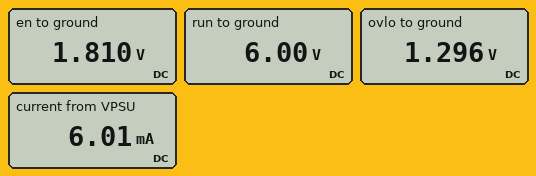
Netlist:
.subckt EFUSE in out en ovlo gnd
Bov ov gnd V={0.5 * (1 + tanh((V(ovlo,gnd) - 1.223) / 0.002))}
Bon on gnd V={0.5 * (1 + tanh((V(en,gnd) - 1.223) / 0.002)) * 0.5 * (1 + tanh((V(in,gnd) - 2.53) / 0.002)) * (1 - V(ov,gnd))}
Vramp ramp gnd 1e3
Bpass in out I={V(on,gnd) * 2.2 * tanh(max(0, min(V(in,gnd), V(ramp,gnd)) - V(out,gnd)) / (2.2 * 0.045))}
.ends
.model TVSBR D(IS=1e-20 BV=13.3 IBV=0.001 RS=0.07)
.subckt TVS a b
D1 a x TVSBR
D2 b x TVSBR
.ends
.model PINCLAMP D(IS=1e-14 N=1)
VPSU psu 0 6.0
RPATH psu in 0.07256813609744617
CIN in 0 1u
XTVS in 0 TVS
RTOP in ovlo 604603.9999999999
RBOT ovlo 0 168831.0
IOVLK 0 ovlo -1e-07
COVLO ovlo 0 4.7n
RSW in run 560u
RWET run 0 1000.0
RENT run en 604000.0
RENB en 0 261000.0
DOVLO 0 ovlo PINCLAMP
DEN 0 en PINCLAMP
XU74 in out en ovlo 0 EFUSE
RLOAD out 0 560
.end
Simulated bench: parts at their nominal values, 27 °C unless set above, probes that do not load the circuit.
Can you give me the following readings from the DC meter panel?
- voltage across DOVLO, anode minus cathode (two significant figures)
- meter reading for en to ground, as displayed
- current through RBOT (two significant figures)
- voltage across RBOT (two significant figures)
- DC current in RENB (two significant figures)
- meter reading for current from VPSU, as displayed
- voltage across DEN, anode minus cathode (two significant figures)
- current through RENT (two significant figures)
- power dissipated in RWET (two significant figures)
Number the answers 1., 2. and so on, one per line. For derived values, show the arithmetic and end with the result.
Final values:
1. 0 V - 1.296 V = -1.3 V
2. 1.810 V
3. (1.296 V) / 168.8 kΩ = 7.7 µA
4. 1.296 V = 1.3 V
5. (1.81 V) / 261 kΩ = 6.9 µA
6. 6.01 mA
7. 0 V - 1.81 V = -1.8 V
8. (6 V - 1.81 V) / 604 kΩ = 6.9 µA
9. (6 V)^2 / 1 kΩ = 36 mW
